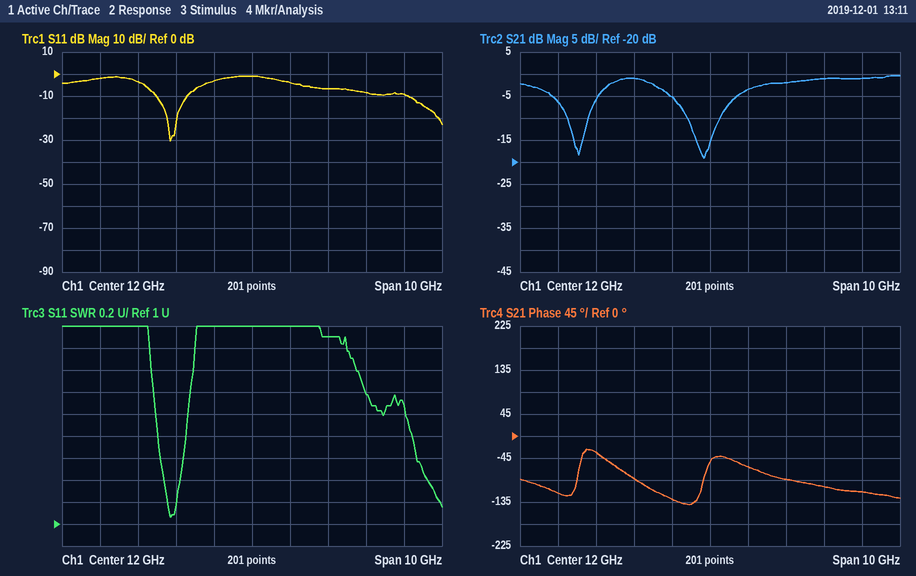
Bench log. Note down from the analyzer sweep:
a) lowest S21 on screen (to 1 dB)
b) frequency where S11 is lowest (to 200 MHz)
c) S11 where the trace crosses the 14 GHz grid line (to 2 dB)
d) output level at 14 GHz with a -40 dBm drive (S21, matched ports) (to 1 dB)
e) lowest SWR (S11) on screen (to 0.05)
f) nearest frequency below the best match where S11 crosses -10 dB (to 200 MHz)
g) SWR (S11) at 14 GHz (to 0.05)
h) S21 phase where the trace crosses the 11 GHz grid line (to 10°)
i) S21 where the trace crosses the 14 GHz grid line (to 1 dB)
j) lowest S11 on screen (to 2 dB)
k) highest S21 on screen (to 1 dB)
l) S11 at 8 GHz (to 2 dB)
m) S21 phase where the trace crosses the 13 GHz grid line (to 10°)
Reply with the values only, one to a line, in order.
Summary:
-19 dB
9.8 GHz
-6 dB
-42 dBm
1.05
9.4 GHz
2.70
-130°
-2 dB
-30 dB
0 dB
-2 dB
-60°
